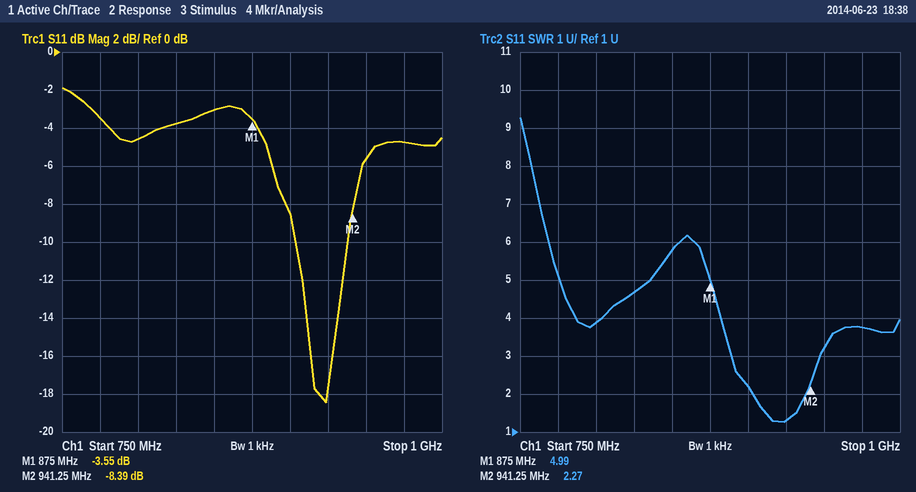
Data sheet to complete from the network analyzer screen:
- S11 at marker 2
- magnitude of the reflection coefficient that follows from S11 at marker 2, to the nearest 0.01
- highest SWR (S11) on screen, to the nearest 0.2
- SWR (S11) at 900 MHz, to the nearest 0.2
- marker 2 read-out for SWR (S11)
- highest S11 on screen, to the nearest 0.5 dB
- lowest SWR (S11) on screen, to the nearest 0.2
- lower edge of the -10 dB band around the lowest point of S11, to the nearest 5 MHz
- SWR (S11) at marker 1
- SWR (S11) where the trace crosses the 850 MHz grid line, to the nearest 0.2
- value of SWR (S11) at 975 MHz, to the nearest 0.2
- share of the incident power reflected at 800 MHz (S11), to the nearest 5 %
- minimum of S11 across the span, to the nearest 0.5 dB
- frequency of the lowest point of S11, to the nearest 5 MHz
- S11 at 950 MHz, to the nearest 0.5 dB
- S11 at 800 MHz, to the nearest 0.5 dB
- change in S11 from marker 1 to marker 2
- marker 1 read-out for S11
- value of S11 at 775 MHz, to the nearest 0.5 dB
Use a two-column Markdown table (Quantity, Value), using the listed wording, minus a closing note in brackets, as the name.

| Quantity | Value |
|---|---|
| S11 at marker 2 | -8.39 dB |
| magnitude of the reflection coefficient that follows from S11 at marker 2, to the nearest 0.01 | 0.38 |
| highest SWR (S11) on screen, to the nearest 0.2 | 9.2 |
| SWR (S11) at 900 MHz, to the nearest 0.2 | 2.2 |
| marker 2 read-out for SWR | 2.27 |
| highest S11 on screen, to the nearest 0.5 dB | -2.0 dB |
| lowest SWR (S11) on screen, to the nearest 0.2 | 1.2 |
| lower edge of the -10 dB band around the lowest point of S11, to the nearest 5 MHz | 905 MHz |
| SWR (S11) at marker 1 | 4.99 |
| SWR (S11) where the trace crosses the 850 MHz grid line, to the nearest 0.2 | 5.8 |
| value of SWR (S11) at 975 MHz, to the nearest 0.2 | 3.8 |
| share of the incident power reflected at 800 MHz (S11), to the nearest 5 % | 35 % |
| minimum of S11 across the span, to the nearest 0.5 dB | -18.5 dB |
| frequency of the lowest point of S11, to the nearest 5 MHz | 925 MHz |
| S11 at 950 MHz, to the nearest 0.5 dB | -5.5 dB |
| S11 at 800 MHz, to the nearest 0.5 dB | -4.5 dB |
| change in S11 from marker 1 to marker 2 | -4.84 dB |
| marker 1 read-out for S11 | -3.55 dB |
| value of S11 at 775 MHz, to the nearest 0.5 dB | -3.5 dB |
